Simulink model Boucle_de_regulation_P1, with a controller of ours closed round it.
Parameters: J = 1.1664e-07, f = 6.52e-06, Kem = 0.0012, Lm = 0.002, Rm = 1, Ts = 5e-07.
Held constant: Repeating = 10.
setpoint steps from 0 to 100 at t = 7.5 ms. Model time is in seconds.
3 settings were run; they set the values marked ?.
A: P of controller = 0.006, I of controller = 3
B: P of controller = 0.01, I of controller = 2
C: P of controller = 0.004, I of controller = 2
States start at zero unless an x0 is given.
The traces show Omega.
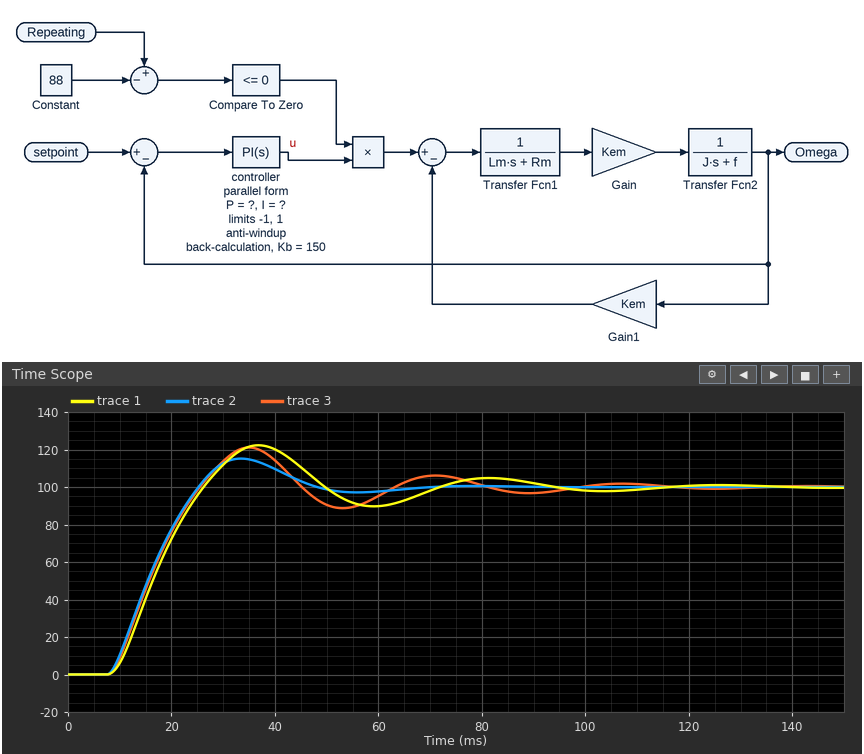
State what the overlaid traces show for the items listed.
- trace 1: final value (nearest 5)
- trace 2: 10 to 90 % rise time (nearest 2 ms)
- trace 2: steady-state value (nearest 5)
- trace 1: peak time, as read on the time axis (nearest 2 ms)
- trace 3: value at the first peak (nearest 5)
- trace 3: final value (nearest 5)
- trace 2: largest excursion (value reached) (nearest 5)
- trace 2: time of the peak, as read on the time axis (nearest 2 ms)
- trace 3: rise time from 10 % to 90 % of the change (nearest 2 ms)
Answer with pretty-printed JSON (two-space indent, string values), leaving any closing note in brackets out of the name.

{
  "trace 1: final value": "100",
  "trace 2: 10 to 90 % rise time": "12 ms",
  "trace 2: steady-state value": "100",
  "trace 1: peak time, as read on the time axis": "36 ms",
  "trace 3: value at the first peak": "120",
  "trace 3: final value": "100",
  "trace 2: largest excursion (value reached)": "115",
  "trace 2: time of the peak, as read on the time axis": "34 ms",
  "trace 3: rise time from 10 % to 90 % of the change": "12 ms"
}
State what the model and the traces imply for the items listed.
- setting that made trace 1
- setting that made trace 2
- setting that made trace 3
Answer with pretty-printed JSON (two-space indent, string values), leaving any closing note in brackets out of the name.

{
  "setting that made trace 1": "C",
  "setting that made trace 2": "B",
  "setting that made trace 3": "A"
}
